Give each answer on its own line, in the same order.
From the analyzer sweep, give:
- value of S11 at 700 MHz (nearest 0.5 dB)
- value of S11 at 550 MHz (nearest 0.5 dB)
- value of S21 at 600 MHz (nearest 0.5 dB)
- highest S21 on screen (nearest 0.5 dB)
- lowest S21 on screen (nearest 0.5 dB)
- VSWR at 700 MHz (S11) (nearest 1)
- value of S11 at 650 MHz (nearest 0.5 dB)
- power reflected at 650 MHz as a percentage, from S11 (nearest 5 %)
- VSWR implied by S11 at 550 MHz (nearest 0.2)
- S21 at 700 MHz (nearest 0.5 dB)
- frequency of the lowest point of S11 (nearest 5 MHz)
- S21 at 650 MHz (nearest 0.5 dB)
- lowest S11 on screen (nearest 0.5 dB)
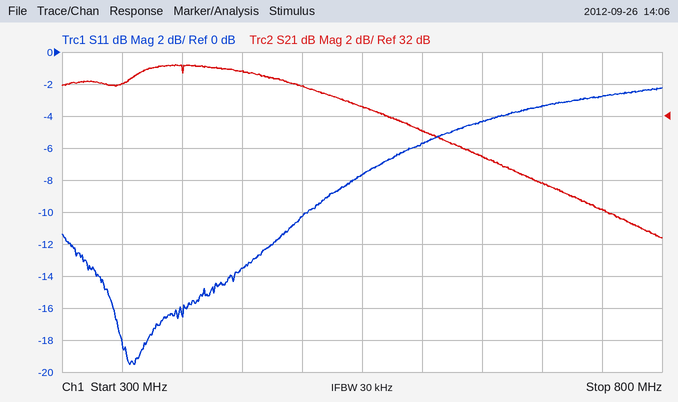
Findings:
-3.5 dB
-7.5 dB
31.0 dB
35.0 dB
24.5 dB
5
-4.5 dB
35 %
2.4
28.0 dB
355 MHz
29.5 dB
-19.5 dB
